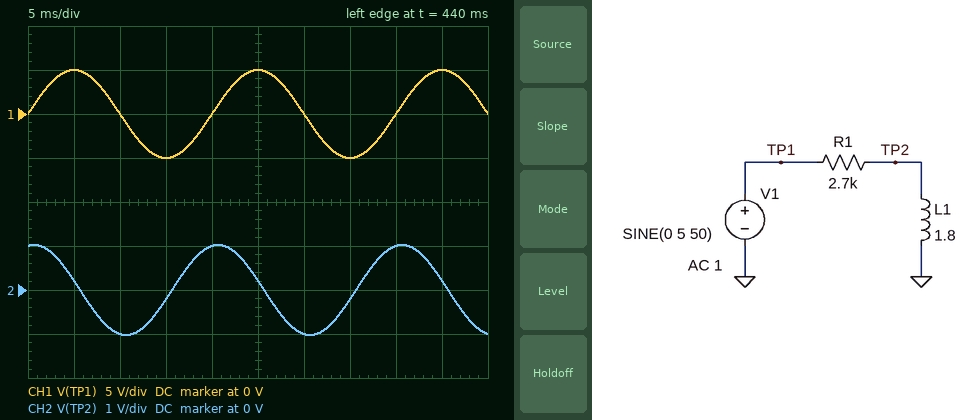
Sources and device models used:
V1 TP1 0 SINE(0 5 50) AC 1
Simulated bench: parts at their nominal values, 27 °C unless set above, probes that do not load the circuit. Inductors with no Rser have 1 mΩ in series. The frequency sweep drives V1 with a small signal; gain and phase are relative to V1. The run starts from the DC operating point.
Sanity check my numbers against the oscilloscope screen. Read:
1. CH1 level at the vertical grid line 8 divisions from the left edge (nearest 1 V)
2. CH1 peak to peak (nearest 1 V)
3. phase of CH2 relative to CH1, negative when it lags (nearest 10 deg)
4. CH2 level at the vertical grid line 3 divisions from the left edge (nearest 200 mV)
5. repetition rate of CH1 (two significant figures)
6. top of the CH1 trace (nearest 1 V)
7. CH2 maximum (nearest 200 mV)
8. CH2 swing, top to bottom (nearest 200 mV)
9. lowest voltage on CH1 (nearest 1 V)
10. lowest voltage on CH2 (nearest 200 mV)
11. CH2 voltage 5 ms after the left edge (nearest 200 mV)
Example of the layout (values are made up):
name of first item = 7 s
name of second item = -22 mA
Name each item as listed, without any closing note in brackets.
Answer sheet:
CH1 level at the vertical grid line 8 divisions from the left edge = 0 V
CH1 peak to peak = 10 V
phase of CH2 relative to CH1, negative when it lags = 80 deg
CH2 level at the vertical grid line 3 divisions from the left edge = -200 mV
repetition rate of CH1 = 50 Hz
top of the CH1 trace = 5 V
CH2 maximum = 1.0 V
CH2 swing, top to bottom = 2.0 V
lowest voltage on CH1 = -5 V
lowest voltage on CH2 = -1.0 V
CH2 voltage 5 ms after the left edge = 200 mV
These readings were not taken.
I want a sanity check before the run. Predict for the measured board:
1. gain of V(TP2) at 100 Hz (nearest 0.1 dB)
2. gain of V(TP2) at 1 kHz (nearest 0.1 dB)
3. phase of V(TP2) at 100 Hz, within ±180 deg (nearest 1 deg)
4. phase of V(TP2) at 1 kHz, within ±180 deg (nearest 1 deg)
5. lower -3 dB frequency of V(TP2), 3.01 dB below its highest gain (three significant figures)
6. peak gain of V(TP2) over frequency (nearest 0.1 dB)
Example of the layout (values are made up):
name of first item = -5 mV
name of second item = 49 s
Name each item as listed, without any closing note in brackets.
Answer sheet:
gain of V(TP2) at 100 Hz = -8.3 dB
gain of V(TP2) at 1 kHz = -0.2 dB
phase of V(TP2) at 100 Hz, within ±180 deg = 67 deg
phase of V(TP2) at 1 kHz, within ±180 deg = 13 deg
lower -3 dB frequency of V(TP2), 3.01 dB below its highest gain = 239 Hz
peak gain of V(TP2) over frequency = 0 dB
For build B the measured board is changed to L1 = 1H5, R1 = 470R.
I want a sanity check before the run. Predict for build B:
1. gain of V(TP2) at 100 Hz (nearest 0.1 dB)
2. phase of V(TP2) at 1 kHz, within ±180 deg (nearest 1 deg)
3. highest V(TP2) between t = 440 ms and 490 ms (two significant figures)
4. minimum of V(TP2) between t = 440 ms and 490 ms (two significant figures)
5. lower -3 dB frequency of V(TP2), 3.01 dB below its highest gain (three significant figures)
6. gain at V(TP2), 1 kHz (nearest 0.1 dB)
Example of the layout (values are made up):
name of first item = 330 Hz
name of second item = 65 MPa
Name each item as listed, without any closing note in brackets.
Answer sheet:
gain of V(TP2) at 100 Hz = -1.0 dB
phase of V(TP2) at 1 kHz, within ±180 deg = 3 deg
highest V(TP2) between t = 440 ms and 490 ms = 3.5 V
minimum of V(TP2) between t = 440 ms and 490 ms = -3.5 V
lower -3 dB frequency of V(TP2), 3.01 dB below its highest gain = 49.9 Hz
gain at V(TP2), 1 kHz = 0 dB
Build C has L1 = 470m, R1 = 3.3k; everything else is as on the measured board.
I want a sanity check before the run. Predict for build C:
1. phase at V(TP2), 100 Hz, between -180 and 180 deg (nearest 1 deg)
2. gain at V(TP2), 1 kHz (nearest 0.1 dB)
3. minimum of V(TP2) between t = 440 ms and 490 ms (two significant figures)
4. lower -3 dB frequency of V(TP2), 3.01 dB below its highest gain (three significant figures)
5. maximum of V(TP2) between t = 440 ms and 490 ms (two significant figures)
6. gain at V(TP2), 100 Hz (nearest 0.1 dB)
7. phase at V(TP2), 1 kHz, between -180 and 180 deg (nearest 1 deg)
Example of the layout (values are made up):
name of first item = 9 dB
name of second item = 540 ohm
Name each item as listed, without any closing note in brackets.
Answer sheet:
phase at V(TP2), 100 Hz, between -180 and 180 deg = 85 deg
gain at V(TP2), 1 kHz = -3.5 dB
minimum of V(TP2) between t = 440 ms and 490 ms = -220 mV
lower -3 dB frequency of V(TP2), 3.01 dB below its highest gain = 1.12 kHz
maximum of V(TP2) between t = 440 ms and 490 ms = 220 mV
gain at V(TP2), 100 Hz = -21.0 dB
phase at V(TP2), 1 kHz, between -180 and 180 deg = 48 deg
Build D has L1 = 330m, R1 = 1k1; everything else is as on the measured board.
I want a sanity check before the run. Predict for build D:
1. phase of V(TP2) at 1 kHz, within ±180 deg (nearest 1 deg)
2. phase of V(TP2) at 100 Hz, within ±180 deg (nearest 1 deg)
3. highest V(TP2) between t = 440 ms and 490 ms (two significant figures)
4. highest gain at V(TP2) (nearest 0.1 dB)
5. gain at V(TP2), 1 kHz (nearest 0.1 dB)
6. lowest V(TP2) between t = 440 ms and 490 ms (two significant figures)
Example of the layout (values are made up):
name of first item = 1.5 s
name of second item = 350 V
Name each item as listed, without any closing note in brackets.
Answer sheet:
phase of V(TP2) at 1 kHz, within ±180 deg = 28 deg
phase of V(TP2) at 100 Hz, within ±180 deg = 79 deg
highest V(TP2) between t = 440 ms and 490 ms = 470 mV
highest gain at V(TP2) = 0 dB
gain at V(TP2), 1 kHz = -1.1 dB
lowest V(TP2) between t = 440 ms and 490 ms = -470 mV
